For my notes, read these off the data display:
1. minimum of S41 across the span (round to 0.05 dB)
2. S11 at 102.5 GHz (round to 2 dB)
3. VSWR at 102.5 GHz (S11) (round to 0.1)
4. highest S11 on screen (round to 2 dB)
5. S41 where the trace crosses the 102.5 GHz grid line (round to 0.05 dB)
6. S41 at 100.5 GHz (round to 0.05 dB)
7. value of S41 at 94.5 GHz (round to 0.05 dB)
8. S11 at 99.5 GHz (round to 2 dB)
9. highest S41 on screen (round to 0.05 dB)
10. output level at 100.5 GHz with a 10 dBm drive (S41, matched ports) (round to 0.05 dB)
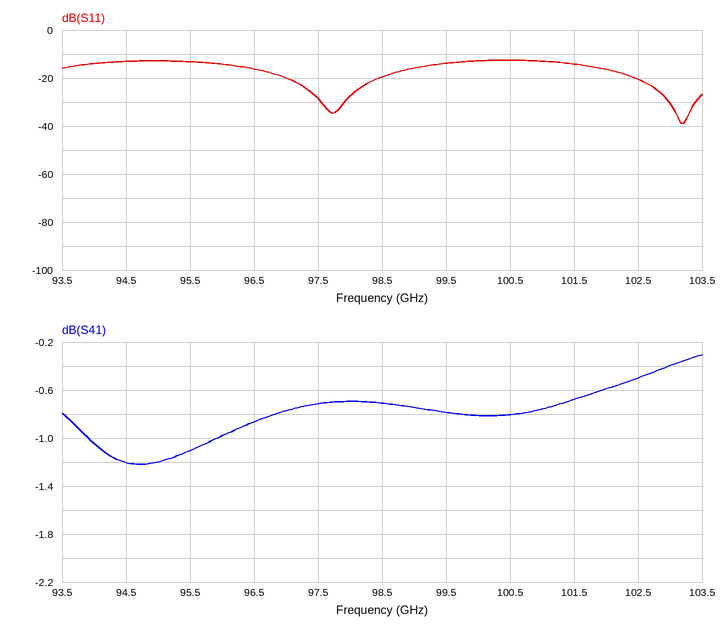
-1.20 dB
-20 dB
1.2
-12 dB
-0.50 dB
-0.80 dB
-1.20 dB
-14 dB
-0.30 dB
9.20 dBm
